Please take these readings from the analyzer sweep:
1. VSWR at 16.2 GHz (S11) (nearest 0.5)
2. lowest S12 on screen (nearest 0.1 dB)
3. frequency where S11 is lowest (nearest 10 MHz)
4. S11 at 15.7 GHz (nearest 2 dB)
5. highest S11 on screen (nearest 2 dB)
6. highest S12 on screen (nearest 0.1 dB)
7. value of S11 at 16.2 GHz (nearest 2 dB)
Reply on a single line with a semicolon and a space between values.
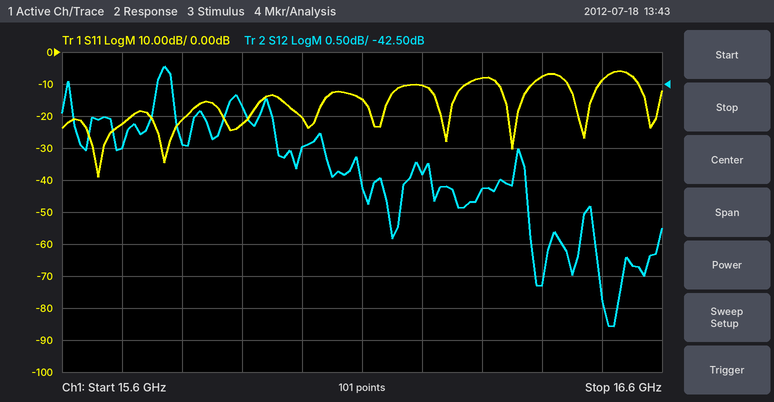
2.0; -46.3 dB; 15.66 GHz; -22 dB; -6 dB; -42.2 dB; -10 dB
